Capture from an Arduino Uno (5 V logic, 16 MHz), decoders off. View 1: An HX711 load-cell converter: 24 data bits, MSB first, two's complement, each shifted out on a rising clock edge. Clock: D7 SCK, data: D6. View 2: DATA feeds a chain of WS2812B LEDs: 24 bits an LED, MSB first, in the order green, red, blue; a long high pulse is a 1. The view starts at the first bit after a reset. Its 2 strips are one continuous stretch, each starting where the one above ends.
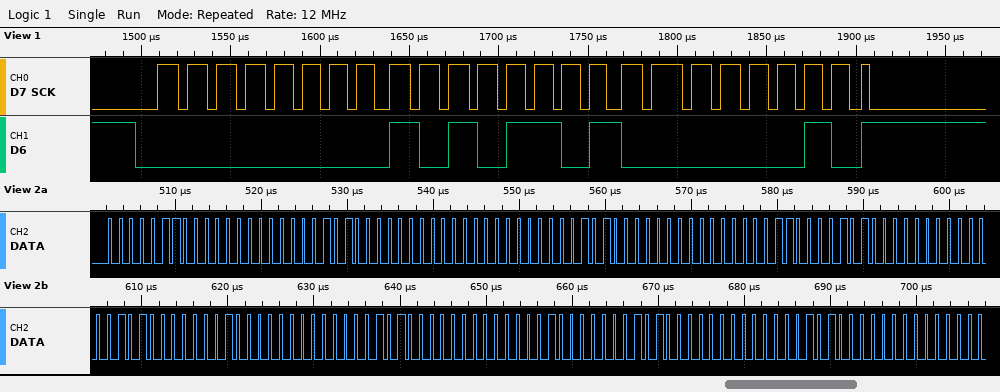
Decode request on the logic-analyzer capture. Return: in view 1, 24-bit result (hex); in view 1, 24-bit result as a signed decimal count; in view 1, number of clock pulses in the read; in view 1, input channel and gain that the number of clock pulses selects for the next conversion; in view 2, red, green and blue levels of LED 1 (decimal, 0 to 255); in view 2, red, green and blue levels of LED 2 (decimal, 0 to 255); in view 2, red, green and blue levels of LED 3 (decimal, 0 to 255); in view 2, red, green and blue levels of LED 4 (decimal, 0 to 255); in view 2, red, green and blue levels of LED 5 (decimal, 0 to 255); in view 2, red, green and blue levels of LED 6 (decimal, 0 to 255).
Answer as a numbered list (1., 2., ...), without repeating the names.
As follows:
1. 0x00AD02
2. 44290
3. 25
4. channel A, gain 128
5. 0, 6, 10
6. 0, 0, 10
7. 3, 0, 10
8. 10, 0, 2
9. 10, 0, 0
10. 10, 8, 0
